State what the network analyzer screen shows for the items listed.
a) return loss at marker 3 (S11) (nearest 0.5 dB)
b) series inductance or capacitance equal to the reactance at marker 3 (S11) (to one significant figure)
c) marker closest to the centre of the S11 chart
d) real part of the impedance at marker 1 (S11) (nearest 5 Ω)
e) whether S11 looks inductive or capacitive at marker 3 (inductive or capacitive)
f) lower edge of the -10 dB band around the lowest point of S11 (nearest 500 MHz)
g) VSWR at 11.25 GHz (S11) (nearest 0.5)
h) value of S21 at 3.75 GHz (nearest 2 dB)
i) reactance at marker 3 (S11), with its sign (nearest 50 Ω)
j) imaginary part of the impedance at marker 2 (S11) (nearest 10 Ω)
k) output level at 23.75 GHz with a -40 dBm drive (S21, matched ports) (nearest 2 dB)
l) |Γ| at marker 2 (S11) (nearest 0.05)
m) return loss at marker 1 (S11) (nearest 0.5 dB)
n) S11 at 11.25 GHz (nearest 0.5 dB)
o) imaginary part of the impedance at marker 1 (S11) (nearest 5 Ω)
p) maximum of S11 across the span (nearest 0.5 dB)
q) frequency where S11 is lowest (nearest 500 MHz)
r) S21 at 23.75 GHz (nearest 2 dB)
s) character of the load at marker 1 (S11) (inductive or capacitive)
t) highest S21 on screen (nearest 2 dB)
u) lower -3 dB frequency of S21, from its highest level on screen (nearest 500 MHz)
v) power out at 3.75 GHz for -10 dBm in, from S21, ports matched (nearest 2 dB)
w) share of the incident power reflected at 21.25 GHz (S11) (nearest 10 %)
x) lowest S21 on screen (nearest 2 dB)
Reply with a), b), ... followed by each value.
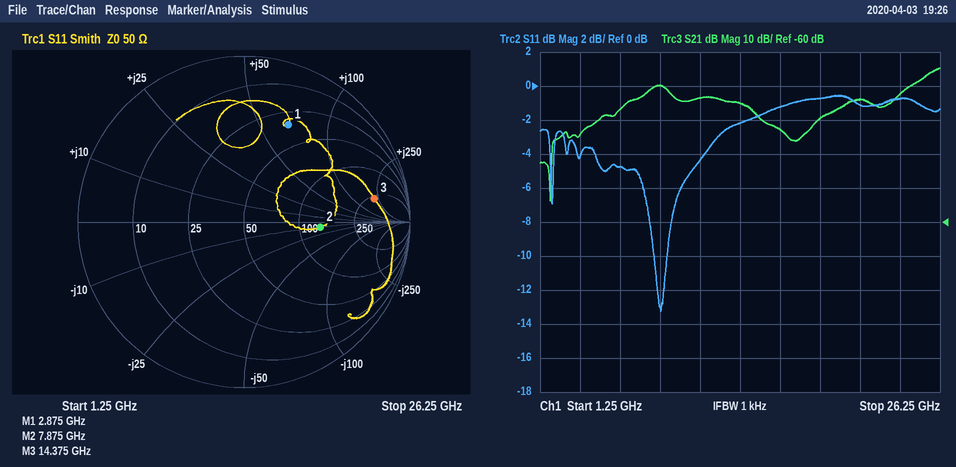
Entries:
a) 2.0 dB
b) 2 nH
c) marker 2
d) 35 Ω
e) inductive
f) 8.5 GHz
g) 4.0
h) -34 dB
i) +200 Ω
j) -10 Ω
k) -62 dBm
l) 0.45
m) 4.0 dB
n) -4.5 dB
o) +65 Ω
p) -0.5 dB
q) 9.0 GHz
r) -22 dB
s) inductive
t) -14 dB
u) 25.0 GHz
v) -44 dBm
w) 80 %
x) -54 dB
